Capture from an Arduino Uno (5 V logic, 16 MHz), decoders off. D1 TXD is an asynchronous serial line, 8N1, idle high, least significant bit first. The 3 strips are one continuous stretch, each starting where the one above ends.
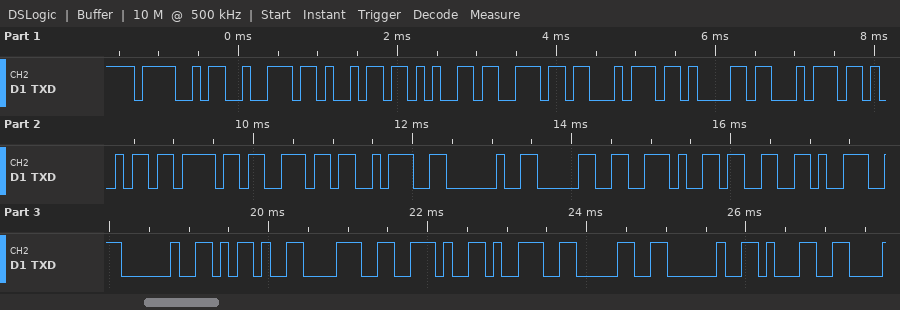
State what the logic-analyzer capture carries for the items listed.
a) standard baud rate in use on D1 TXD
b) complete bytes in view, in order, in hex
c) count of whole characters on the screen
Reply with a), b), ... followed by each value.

a) 9600 baud
b) 4F 72 69 65 6E 74 61 74 69 6F 6E 3A 20 30 2E 33 39 20 2D 38 2E 39 30 20 31
c) 25
